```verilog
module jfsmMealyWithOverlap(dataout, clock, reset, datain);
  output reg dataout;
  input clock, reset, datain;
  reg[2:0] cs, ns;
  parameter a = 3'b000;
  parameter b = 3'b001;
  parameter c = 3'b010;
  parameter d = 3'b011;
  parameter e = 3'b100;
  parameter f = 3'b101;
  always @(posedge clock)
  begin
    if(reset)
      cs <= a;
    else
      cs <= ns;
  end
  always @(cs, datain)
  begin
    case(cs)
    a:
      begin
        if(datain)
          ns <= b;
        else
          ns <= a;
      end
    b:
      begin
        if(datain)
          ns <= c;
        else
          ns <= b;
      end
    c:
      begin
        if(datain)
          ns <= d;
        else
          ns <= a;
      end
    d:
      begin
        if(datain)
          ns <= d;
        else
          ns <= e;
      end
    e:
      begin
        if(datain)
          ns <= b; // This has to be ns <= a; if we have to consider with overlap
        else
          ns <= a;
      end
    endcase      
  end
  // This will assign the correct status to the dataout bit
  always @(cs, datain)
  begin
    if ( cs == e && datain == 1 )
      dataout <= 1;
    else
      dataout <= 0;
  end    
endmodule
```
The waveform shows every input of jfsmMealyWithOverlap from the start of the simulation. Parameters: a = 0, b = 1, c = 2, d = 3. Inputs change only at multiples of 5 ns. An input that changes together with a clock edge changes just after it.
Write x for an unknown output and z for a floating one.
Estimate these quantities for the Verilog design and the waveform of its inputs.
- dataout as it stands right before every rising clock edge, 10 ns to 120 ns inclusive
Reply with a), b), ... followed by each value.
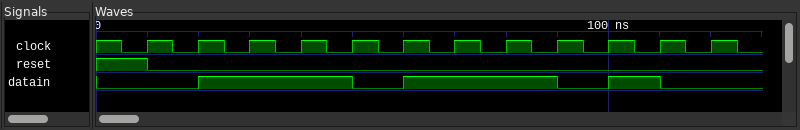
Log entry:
a) 0 0 0 0 0 0 1 0 0 0 1 0
